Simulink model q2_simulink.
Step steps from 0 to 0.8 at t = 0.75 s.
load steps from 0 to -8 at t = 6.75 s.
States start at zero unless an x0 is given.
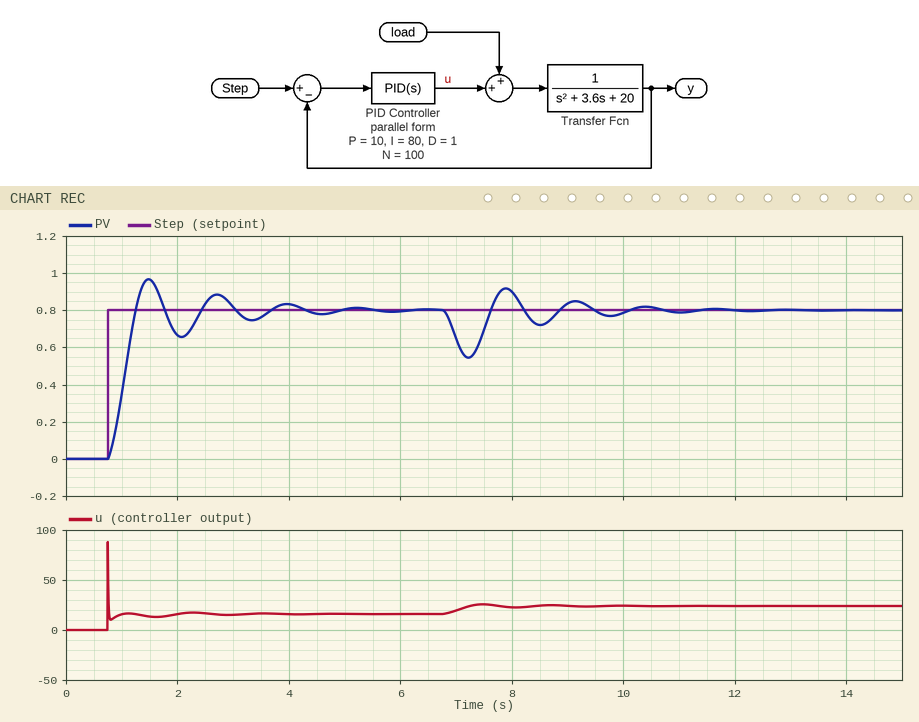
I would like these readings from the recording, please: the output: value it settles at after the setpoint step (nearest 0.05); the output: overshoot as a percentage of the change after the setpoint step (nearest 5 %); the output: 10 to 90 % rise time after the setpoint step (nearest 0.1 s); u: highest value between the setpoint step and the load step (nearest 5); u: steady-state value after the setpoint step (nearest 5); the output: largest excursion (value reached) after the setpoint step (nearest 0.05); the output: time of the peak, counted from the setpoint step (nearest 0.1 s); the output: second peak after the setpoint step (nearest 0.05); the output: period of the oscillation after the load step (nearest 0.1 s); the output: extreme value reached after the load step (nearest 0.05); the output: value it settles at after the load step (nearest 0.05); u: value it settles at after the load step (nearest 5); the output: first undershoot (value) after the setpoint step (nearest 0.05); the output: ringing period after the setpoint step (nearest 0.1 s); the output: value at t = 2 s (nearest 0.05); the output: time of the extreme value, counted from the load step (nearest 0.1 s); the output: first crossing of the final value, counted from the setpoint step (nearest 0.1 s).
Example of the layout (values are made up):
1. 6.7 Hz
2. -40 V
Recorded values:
1. 0.80
2. 20 %
3. 0.4 s
4. 90
5. 15
6. 0.95
7. 0.7 s
8. 0.90
9. 1.3 s
10. 0.55
11. 0.80
12. 25
13. 0.65
14. 1.2 s
15. 0.65
16. 0.5 s
17. 0.5 s
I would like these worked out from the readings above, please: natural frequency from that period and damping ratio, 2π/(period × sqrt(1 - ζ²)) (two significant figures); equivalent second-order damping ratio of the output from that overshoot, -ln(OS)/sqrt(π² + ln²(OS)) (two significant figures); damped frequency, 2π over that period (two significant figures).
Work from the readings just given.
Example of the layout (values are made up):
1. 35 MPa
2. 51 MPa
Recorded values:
1. 5.9 rad/s
2. 0.46
3. 5.2 rad/s
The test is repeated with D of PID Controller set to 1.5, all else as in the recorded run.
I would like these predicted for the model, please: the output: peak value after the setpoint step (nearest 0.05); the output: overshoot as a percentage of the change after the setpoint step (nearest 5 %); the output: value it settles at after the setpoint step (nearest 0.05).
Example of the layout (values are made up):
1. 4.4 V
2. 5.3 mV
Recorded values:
1. 0.90
2. 15 %
3. 0.80
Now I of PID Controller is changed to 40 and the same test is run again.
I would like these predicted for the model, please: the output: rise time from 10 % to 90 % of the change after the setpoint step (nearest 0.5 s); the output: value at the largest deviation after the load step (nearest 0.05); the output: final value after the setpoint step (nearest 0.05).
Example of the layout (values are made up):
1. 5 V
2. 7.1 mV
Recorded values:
1. 1.5 s
2. 0.50
3. 0.80
